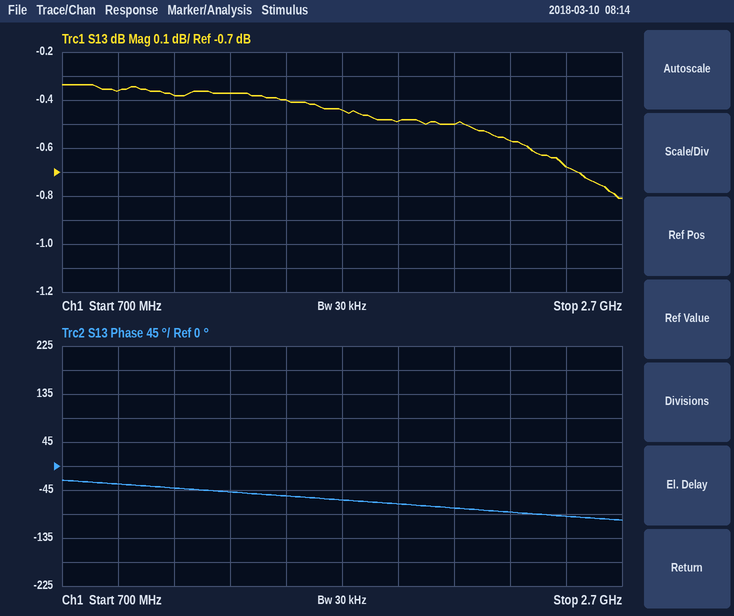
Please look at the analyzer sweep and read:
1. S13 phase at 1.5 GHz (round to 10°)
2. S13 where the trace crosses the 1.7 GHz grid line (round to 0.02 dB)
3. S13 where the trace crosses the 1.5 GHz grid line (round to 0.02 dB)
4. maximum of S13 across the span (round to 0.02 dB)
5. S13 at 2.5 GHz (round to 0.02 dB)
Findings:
-60°
-0.44 dB
-0.40 dB
-0.34 dB
-0.68 dB
